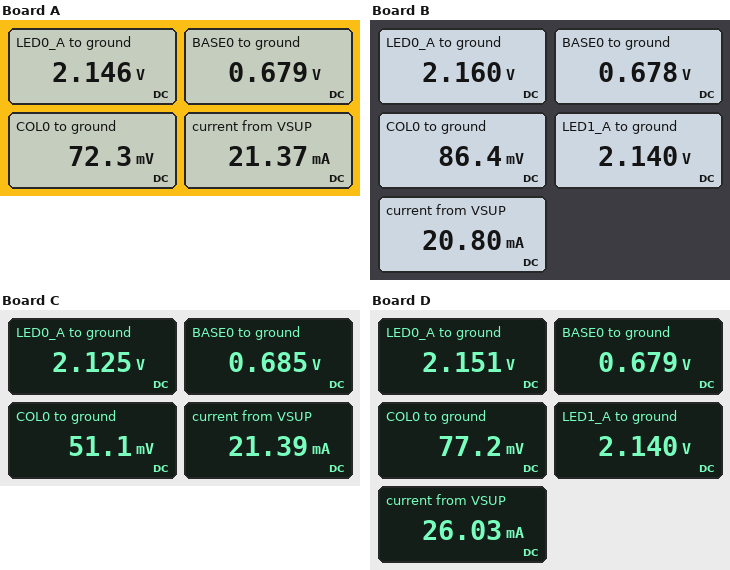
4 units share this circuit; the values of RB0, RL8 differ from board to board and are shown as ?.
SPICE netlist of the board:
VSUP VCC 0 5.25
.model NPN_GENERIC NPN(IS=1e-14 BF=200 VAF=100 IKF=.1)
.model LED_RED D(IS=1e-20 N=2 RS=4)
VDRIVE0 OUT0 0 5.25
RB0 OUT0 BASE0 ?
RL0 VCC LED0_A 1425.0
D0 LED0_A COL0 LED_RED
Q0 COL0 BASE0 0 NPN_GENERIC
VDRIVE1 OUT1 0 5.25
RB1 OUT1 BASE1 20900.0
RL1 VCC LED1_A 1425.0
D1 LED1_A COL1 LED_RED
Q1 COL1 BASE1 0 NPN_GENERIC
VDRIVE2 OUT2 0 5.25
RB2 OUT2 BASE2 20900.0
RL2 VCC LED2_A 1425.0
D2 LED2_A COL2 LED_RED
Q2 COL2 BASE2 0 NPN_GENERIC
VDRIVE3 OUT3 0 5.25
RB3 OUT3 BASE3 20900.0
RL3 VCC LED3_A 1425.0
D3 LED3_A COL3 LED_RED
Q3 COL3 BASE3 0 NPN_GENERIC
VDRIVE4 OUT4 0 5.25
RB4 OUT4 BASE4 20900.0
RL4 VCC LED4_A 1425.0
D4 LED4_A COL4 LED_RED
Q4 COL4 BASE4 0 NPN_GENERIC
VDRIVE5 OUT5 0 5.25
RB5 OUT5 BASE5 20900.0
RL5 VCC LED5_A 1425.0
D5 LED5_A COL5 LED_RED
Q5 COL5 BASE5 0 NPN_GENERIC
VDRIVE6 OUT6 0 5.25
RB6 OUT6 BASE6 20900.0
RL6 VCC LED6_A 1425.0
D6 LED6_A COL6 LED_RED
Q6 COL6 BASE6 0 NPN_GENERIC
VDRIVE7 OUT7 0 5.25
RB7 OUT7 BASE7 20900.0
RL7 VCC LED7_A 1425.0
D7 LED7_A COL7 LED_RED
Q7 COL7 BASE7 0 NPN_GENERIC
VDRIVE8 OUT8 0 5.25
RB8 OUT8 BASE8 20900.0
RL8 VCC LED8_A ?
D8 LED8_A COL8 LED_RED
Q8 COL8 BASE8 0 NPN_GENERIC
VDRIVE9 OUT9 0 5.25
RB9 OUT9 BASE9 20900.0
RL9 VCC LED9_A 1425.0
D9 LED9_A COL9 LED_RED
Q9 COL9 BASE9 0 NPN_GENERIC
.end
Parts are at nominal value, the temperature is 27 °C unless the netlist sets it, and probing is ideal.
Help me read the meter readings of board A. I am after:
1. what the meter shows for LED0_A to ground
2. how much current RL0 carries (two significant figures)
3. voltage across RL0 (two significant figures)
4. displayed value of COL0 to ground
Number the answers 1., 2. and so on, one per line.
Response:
1. 2.146 V
2. 2.2 mA
3. 3.1 V
4. 72.3 mV
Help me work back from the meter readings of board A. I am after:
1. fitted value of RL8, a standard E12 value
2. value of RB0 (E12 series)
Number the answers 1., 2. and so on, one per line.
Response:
1. 1.8 kΩ
2. 27 kΩ
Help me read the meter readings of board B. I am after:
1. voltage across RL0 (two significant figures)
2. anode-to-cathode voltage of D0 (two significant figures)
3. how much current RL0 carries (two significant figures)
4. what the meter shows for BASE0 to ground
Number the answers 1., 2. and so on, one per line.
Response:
1. 3.1 V
2. 2.1 V
3. 2.2 mA
4. 0.678 V
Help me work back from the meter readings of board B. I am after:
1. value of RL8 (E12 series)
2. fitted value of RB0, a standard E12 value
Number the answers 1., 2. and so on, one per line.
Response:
1. 2.7 kΩ
2. 47 kΩ
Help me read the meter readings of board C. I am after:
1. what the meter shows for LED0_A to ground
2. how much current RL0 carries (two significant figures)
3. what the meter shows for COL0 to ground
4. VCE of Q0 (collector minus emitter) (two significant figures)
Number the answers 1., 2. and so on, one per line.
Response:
1. 2.125 V
2. 2.2 mA
3. 51.1 mV
4. 51 mV
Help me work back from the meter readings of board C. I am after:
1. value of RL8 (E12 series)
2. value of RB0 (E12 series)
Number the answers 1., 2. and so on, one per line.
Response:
1. 1.8 kΩ
2. 10 kΩ
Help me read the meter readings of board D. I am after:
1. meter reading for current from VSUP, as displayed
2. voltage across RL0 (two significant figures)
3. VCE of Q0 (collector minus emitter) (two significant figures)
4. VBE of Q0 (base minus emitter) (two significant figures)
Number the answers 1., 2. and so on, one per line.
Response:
1. 26.03 mA
2. 3.1 V
3. 77 mV
4. 680 mV
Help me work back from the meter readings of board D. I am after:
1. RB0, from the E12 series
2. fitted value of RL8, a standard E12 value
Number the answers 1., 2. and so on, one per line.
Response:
1. 33 kΩ
2. 470 Ω
